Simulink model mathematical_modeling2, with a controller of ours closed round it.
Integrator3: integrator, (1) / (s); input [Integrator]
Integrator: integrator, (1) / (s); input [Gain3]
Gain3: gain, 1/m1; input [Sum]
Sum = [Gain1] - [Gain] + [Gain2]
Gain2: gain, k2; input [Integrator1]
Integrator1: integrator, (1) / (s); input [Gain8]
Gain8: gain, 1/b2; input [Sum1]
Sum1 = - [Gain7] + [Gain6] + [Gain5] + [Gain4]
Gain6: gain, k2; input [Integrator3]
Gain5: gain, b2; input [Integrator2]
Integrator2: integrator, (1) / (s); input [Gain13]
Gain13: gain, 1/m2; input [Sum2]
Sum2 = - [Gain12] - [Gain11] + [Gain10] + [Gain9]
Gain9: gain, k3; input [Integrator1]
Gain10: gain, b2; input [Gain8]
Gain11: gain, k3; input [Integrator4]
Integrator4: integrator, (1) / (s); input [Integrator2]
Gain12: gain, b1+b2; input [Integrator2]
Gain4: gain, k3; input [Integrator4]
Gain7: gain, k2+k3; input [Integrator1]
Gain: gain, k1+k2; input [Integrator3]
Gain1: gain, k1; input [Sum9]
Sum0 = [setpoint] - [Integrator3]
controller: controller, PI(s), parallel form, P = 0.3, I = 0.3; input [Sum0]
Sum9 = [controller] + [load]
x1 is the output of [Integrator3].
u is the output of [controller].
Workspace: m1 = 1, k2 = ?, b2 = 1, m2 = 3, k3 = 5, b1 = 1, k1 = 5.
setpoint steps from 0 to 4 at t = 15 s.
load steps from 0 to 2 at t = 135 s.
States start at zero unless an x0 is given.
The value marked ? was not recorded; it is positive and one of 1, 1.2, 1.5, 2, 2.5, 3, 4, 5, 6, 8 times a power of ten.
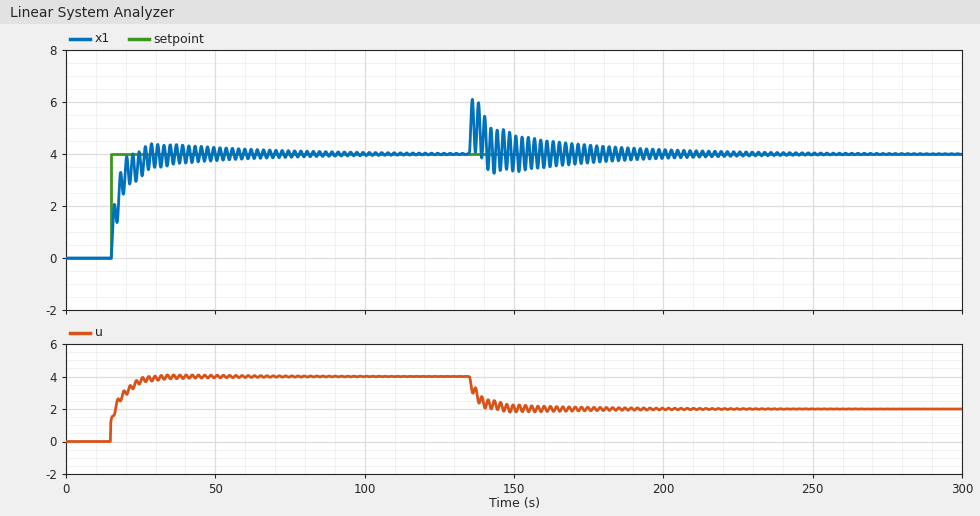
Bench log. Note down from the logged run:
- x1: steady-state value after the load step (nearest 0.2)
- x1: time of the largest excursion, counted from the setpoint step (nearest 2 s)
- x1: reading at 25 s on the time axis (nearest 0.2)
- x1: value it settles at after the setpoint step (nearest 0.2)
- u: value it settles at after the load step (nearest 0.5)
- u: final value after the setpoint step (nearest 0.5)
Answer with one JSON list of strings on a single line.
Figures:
["4.0", "14 s", "3.6", "4.0", "2.0", "4.0"]
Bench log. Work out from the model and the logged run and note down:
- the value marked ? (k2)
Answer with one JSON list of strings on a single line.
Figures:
["4"]
